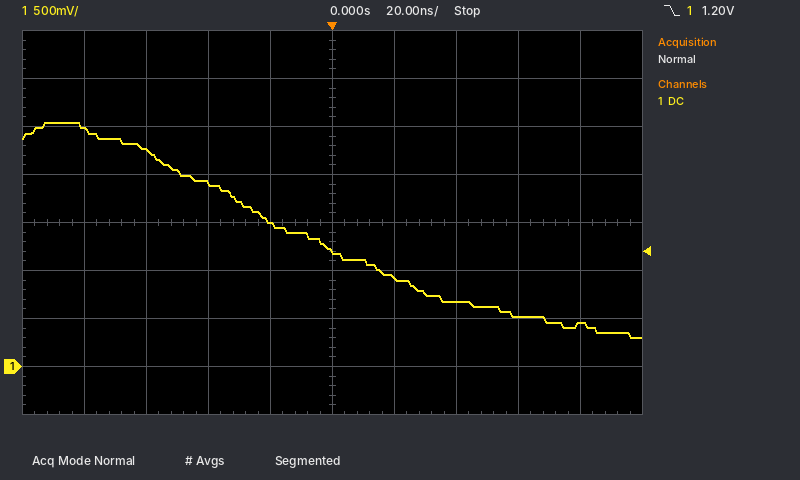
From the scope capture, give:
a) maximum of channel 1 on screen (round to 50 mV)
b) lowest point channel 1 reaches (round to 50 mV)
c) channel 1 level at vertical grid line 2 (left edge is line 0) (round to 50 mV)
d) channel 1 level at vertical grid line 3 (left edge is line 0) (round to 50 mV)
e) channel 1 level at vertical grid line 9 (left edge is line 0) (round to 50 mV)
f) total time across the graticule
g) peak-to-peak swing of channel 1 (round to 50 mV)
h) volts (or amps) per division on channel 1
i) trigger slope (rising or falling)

2.55 V
300 mV
2.25 V
1.90 V
450 mV
200 ns
2.25 V
500 mV
falling
